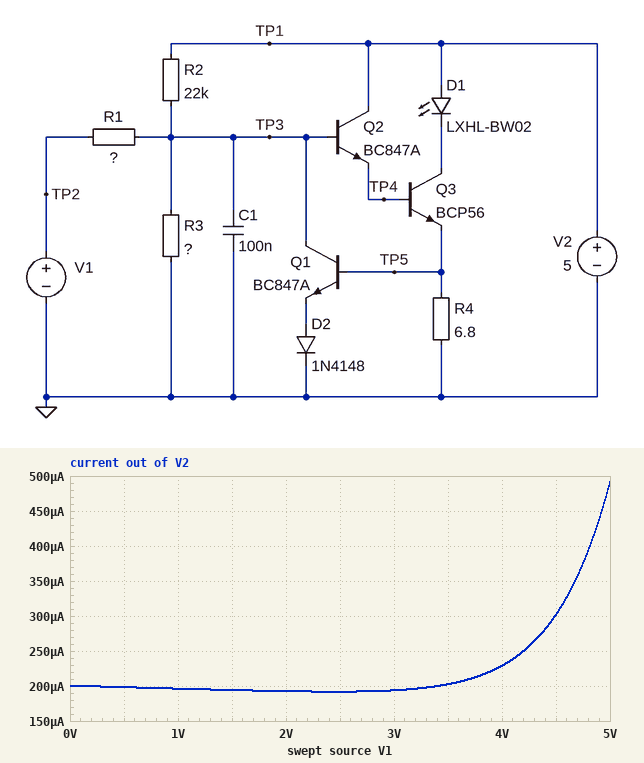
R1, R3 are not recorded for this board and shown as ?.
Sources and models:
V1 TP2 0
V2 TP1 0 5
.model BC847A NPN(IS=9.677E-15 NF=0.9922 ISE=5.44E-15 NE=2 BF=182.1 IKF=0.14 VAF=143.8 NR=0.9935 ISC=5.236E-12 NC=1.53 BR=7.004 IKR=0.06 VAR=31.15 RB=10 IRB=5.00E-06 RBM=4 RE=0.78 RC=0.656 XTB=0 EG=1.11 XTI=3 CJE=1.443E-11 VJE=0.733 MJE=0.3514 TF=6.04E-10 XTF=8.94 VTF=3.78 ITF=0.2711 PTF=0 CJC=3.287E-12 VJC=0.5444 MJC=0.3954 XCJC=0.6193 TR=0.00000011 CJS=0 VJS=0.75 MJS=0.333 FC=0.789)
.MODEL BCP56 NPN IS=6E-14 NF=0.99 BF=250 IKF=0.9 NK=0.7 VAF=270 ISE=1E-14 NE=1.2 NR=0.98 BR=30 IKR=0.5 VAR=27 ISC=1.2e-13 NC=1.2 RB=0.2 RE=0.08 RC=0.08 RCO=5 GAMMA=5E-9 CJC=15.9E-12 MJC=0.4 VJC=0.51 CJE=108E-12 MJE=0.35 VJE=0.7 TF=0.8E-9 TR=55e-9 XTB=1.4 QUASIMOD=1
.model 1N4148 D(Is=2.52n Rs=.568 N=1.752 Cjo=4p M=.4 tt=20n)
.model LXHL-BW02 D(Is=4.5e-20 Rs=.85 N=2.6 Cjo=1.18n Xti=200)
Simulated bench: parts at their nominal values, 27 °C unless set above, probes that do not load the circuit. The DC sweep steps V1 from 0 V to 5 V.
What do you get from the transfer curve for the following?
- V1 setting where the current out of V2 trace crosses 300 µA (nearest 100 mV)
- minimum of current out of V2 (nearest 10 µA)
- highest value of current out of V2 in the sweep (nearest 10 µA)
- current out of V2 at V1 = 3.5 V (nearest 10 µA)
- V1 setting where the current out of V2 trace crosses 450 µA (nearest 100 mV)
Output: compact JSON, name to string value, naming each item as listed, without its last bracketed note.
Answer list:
{"V1 setting where the current out of V2 trace crosses 300 µA": "4.5 V", "minimum of current out of V2": "190 µA", "highest value of current out of V2 in the sweep": "490 µA", "current out of V2 at V1 = 3.5 V": "200 µA", "V1 setting where the current out of V2 trace crosses 450 µA": "4.9 V"}
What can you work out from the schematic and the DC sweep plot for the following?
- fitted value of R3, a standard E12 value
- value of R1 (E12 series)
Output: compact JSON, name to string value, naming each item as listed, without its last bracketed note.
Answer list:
{"fitted value of R3, a standard E12 value": "3.3 kΩ", "value of R1": "27 kΩ"}
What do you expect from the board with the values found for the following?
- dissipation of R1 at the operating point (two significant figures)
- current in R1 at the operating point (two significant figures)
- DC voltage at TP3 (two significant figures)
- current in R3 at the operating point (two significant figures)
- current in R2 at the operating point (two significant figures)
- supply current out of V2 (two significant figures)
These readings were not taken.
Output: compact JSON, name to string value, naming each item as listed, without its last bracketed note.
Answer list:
{"dissipation of R1 at the operating point": "13 µW", "current in R1 at the operating point": "22 µA", "DC voltage at TP3": "590 mV", "current in R3 at the operating point": "180 µA", "current in R2 at the operating point": "200 µA", "supply current out of V2": "200 µA"}
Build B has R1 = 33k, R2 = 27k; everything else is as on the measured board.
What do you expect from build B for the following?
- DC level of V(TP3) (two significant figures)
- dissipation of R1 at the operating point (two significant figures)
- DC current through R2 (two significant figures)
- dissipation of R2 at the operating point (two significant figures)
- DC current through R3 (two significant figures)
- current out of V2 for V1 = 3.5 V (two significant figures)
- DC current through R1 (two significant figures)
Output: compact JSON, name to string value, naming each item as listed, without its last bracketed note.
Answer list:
{"DC level of V(TP3)": "500 mV", "dissipation of R1 at the operating point": "7.6 µW", "DC current through R2": "170 µA", "dissipation of R2 at the operating point": "750 µW", "DC current through R3": "150 µA", "current out of V2 for V1 = 3.5 V": "160 µA", "DC current through R1": "15 µA"}
